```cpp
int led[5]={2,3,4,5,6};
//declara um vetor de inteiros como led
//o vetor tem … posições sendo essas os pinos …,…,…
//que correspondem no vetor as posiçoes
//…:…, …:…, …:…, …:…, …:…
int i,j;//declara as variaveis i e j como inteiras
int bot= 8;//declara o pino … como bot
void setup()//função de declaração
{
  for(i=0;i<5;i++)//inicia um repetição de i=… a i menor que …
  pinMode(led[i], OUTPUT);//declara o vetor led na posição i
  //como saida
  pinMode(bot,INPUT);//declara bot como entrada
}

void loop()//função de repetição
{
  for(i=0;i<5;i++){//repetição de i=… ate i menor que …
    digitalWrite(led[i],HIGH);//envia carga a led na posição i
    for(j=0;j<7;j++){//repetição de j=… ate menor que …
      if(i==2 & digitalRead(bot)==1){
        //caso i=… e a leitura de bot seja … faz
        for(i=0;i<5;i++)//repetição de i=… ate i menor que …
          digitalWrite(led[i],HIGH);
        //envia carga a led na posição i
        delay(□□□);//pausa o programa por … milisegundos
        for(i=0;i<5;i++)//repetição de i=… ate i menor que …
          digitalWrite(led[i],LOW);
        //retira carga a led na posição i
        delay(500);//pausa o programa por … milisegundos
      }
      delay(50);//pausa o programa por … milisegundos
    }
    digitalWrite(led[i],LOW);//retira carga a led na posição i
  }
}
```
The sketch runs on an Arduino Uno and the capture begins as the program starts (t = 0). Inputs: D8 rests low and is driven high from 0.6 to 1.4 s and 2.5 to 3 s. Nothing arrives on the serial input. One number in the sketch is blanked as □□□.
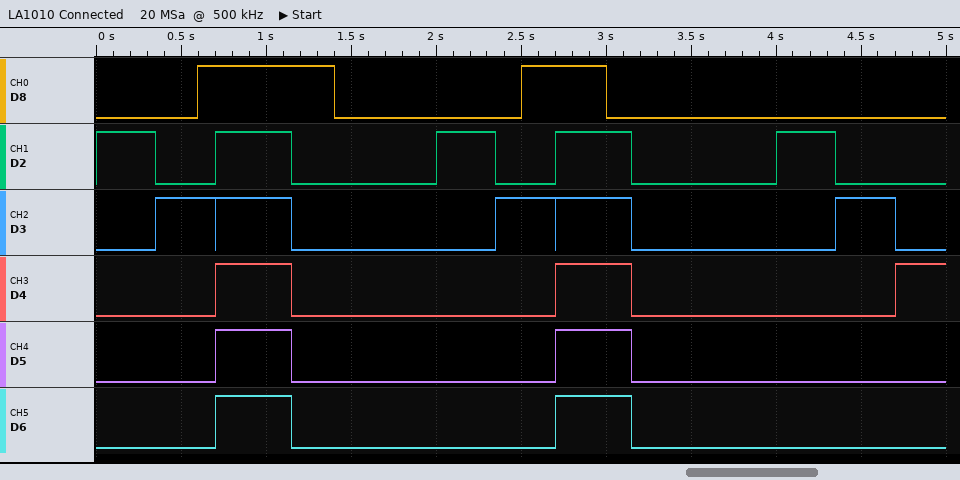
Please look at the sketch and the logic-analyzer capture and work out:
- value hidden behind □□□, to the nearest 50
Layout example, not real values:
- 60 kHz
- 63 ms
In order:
- 450
